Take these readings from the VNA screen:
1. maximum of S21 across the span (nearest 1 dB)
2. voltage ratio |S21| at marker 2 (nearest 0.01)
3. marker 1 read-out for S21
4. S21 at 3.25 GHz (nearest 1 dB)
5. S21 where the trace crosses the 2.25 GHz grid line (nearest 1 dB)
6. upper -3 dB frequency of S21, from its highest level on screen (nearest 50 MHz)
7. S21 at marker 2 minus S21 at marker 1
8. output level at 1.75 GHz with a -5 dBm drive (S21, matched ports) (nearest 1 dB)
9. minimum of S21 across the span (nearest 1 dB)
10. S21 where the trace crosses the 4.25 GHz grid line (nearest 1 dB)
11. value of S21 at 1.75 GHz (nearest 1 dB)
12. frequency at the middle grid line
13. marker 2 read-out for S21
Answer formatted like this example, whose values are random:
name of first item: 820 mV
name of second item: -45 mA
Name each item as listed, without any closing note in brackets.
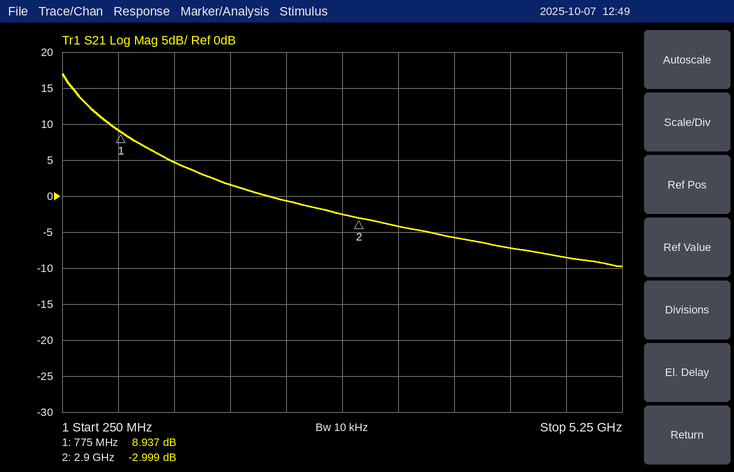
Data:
maximum of S21 across the span: 17 dB
voltage ratio |S21| at marker 2: 0.71
marker 1 read-out for S21: 8.937 dB
S21 at 3.25 GHz: -4 dB
S21 where the trace crosses the 2.25 GHz grid line: -1 dB
upper -3 dB frequency of S21, from its highest level on screen: 400 MHz
S21 at marker 2 minus S21 at marker 1: -11.936 dB
output level at 1.75 GHz with a -5 dBm drive (S21, matched ports): -3 dBm
minimum of S21 across the span: -10 dB
S21 where the trace crosses the 4.25 GHz grid line: -7 dB
value of S21 at 1.75 GHz: 2 dB
frequency at the middle grid line: 2.75 GHz
marker 2 read-out for S21: -2.999 dB
